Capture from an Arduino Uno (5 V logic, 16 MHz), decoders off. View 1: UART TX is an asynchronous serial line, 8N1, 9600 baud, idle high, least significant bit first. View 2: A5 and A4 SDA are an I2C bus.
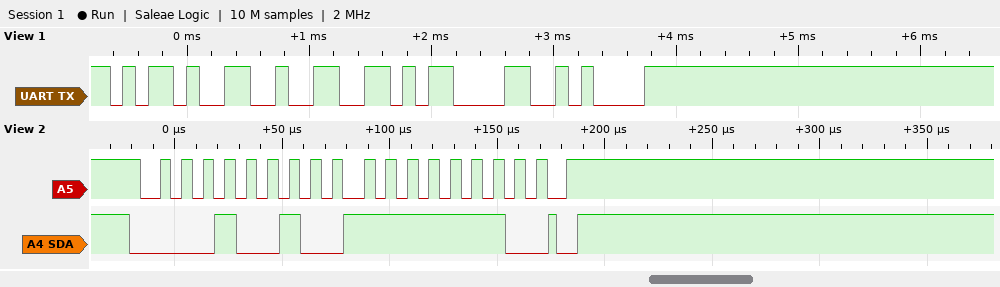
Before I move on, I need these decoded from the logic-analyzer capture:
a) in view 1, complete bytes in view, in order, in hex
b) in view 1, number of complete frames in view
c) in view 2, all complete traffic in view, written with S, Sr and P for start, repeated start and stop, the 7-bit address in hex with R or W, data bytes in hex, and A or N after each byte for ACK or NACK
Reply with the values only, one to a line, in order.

0x2D 0x32 0x0D 0x0A
4
S 09W A FE A P
